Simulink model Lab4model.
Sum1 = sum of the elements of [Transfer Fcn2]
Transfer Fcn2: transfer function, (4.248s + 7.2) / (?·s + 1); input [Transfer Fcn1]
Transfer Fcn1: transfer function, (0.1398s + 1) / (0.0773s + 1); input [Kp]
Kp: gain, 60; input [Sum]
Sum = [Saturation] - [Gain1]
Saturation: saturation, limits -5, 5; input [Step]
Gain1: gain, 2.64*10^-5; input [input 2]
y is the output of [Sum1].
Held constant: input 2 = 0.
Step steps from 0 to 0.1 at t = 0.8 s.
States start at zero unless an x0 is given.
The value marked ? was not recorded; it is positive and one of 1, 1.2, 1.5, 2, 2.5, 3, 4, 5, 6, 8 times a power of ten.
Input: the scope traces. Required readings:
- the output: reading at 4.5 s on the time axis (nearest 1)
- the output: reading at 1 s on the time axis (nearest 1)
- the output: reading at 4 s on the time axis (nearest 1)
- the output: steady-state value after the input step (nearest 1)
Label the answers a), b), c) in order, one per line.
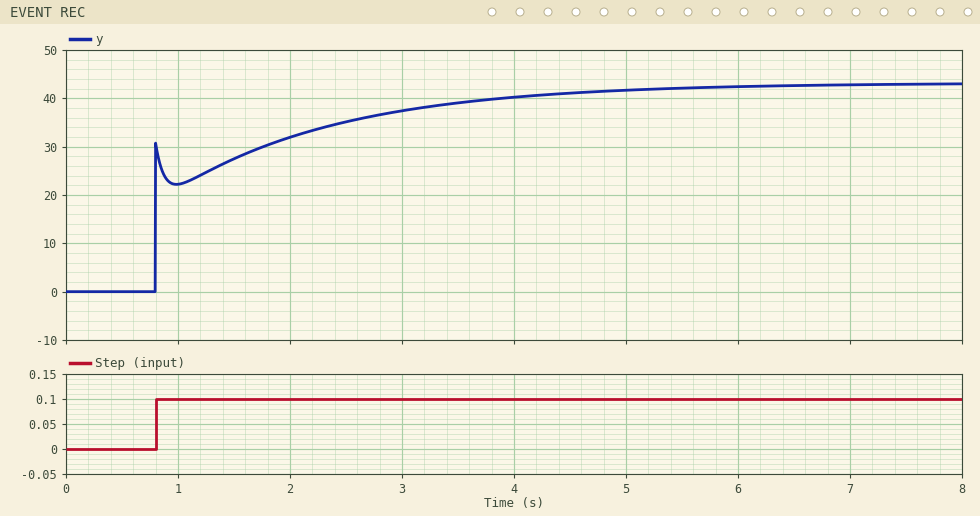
a) 41
b) 22
c) 40
d) 43
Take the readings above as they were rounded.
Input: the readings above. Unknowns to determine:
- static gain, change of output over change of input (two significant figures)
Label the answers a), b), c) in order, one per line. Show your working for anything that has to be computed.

a) (43 - 0) / (0.1 - 0) = 430
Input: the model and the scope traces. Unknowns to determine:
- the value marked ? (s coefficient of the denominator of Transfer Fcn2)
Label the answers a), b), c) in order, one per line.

a) 1.5
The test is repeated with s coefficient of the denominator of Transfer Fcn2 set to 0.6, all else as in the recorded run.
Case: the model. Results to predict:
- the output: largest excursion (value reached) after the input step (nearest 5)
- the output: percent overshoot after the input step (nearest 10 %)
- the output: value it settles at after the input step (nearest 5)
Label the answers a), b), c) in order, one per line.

a) 75
b) 80 %
c) 45
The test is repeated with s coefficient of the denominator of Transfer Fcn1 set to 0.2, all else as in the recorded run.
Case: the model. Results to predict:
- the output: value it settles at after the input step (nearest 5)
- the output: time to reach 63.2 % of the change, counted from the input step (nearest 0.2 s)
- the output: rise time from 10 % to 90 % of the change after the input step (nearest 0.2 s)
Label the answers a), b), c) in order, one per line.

a) 45
b) 0.8 s
c) 2.8 s
